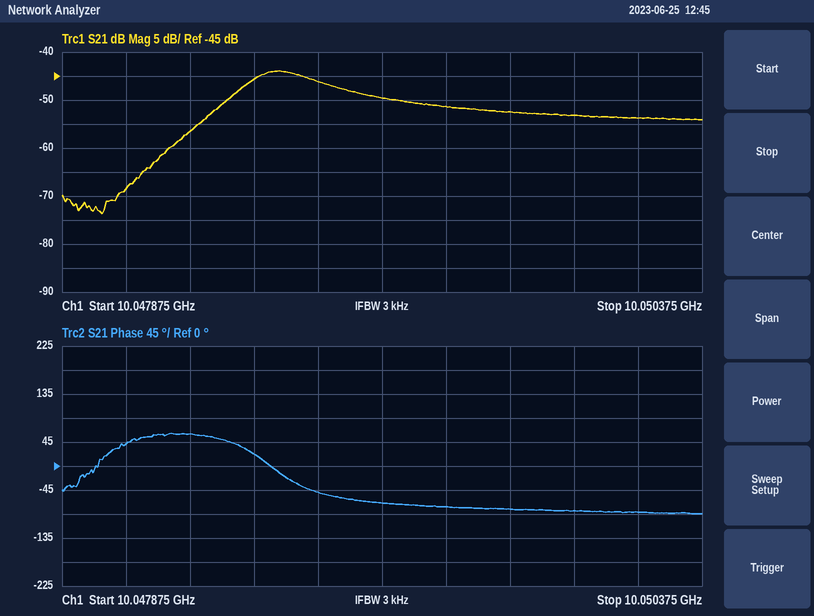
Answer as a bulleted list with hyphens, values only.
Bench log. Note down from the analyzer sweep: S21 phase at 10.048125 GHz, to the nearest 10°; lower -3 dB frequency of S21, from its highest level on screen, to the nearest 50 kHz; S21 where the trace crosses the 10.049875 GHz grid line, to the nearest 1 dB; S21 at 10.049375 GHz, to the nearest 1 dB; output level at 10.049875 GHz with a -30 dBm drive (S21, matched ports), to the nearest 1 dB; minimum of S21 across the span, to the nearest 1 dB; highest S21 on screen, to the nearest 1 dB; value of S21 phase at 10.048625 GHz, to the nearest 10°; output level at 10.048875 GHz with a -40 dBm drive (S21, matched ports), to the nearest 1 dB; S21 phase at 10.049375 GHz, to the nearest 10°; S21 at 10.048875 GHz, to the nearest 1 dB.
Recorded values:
- 40°
- 10.04860 GHz
- -53 dB
- -51 dB
- -83 dBm
- -74 dB
- -44 dB
- 20°
- -86 dBm
- -80°
- -46 dB
